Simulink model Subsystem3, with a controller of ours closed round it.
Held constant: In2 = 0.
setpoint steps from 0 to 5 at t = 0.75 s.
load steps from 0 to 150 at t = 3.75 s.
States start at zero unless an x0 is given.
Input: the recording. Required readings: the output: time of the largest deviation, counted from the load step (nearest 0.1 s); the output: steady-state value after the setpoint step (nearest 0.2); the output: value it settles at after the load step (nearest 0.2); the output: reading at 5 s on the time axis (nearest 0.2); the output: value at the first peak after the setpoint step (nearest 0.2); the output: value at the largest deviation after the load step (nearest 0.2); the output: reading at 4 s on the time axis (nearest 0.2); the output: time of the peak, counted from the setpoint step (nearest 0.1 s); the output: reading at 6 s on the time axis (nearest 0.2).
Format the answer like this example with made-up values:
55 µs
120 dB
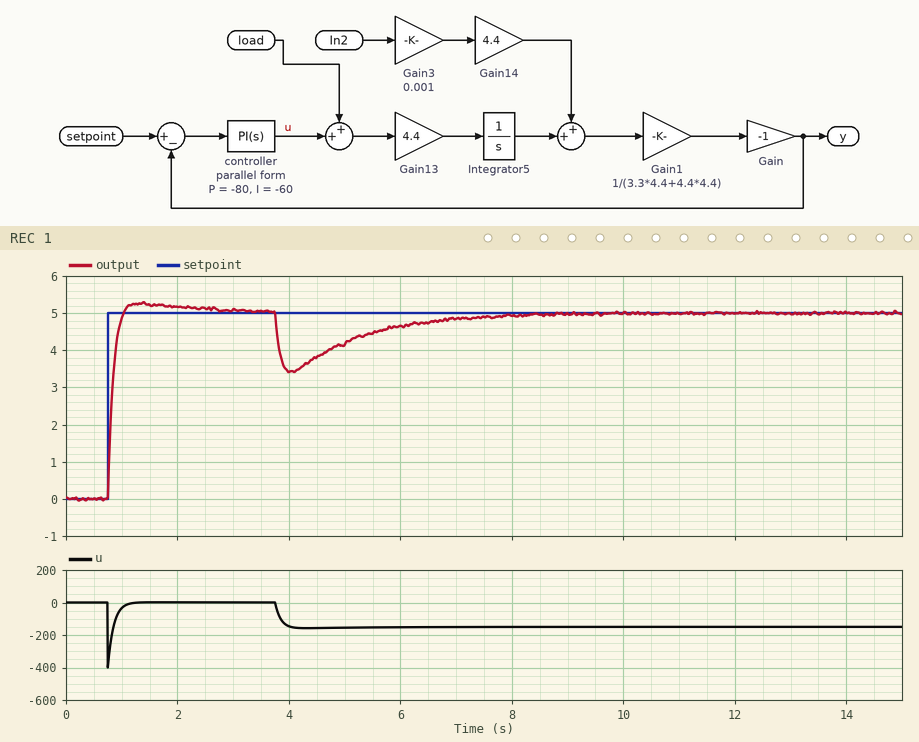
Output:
0.3 s
5.0
5.0
4.2
5.2
3.4
3.4
0.6 s
4.6
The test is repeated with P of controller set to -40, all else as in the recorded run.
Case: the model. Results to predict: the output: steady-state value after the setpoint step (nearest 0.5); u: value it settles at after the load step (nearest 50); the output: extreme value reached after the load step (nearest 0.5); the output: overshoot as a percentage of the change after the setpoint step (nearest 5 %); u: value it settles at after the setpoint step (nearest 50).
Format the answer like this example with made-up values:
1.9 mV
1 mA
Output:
5.0
-150
2.5
15 %
0
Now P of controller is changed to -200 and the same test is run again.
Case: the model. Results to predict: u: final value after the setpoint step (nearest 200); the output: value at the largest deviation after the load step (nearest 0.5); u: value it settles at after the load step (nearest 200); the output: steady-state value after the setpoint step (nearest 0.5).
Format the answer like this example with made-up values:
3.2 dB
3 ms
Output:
0
4.5
-200
5.0
